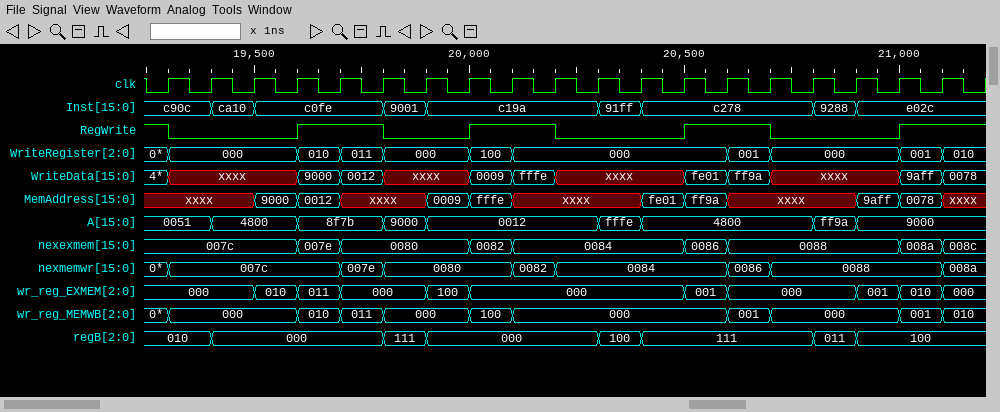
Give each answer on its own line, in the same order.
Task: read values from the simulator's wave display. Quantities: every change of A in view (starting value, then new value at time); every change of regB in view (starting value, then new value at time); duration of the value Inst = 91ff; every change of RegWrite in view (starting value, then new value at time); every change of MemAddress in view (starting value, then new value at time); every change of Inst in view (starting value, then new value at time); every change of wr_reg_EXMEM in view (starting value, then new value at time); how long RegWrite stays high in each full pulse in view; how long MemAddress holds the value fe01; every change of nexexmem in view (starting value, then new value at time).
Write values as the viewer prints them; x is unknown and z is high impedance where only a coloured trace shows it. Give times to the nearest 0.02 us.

0051, 4800 at 19.4 us, 8f7b at 19.6 us, 9000 at 19.8 us, 0012 at 19.9 us, fffe at 20.3 us, 4800 at 20.4 us, ff9a at 20.8 us, 9000 at 20.9 us
010, 000 at 19.4 us, 111 at 19.8 us, 000 at 19.9 us, 100 at 20.3 us, 111 at 20.4 us, 011 at 20.8 us, 100 at 20.9 us
0.1 us
1, 0 at 19.3 us, 1 at 19.6 us, 0 at 19.8 us, 1 at 20 us, 0 at 20.2 us, 1 at 20.5 us, 0 at 20.7 us, 1 at 21 us
xxxx, 9000 at 19.5 us, 0012 at 19.6 us, xxxx at 19.7 us, 0009 at 19.9 us, fffe at 20 us, xxxx at 20.1 us, fe01 at 20.4 us, ff9a at 20.5 us, xxxx at 20.6 us, 9aff at 20.9 us, 0078 at 21 us, xxxx at 21.1 us
c90c, ca10 at 19.4 us, c0fe at 19.5 us, 9001 at 19.8 us, c19a at 19.9 us, 91ff at 20.3 us, c278 at 20.4 us, 9288 at 20.8 us, e02c at 20.9 us
000, 010 at 19.5 us, 011 at 19.6 us, 000 at 19.7 us, 100 at 19.9 us, 000 at 20 us, 001 at 20.5 us, 000 at 20.6 us, 001 at 20.9 us, 010 at 21 us, 000 at 21.1 us
0.2 us, 0.2 us, 0.2 us
0.1 us
007c, 007e at 19.6 us, 0080 at 19.7 us, 0082 at 20 us, 0084 at 20.1 us, 0086 at 20.5 us, 0088 at 20.6 us, 008a at 21 us, 008c at 21.1 us
